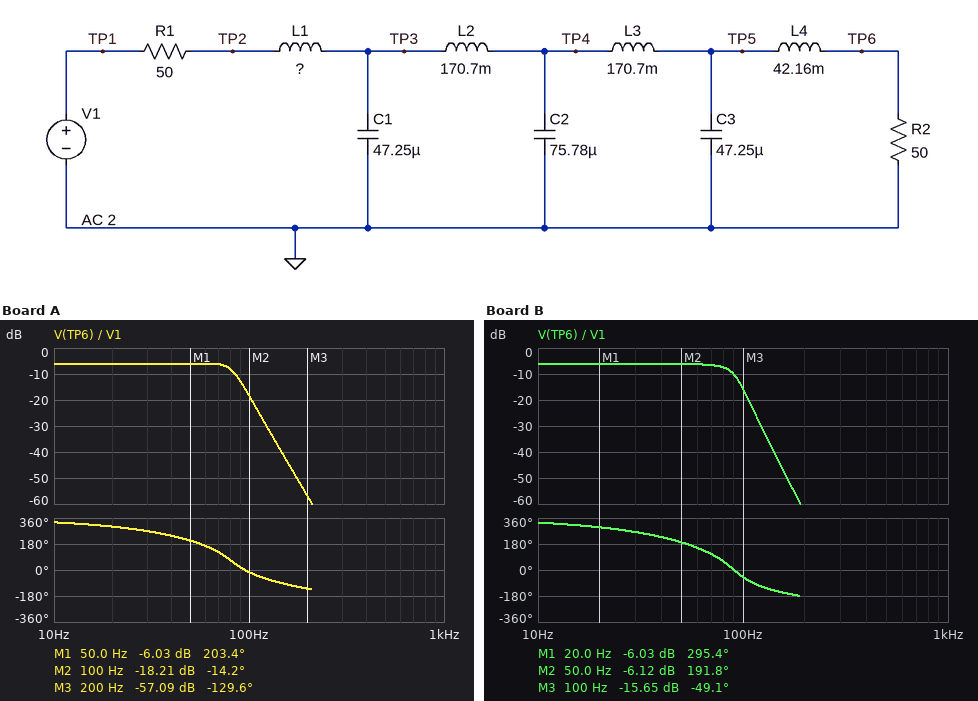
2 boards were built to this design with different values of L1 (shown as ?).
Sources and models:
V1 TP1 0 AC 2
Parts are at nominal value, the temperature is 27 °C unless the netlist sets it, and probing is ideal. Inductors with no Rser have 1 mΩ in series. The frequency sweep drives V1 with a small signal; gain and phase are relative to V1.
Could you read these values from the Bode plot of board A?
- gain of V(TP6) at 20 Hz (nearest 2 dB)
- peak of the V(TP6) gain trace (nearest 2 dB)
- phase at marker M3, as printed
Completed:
-6 dB
-6 dB
-129.6 deg
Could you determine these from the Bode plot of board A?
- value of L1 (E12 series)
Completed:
18 mH
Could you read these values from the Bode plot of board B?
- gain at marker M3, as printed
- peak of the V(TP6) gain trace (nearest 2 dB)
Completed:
-15.65 dB
-6 dB
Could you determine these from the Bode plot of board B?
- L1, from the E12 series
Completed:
82 mH
